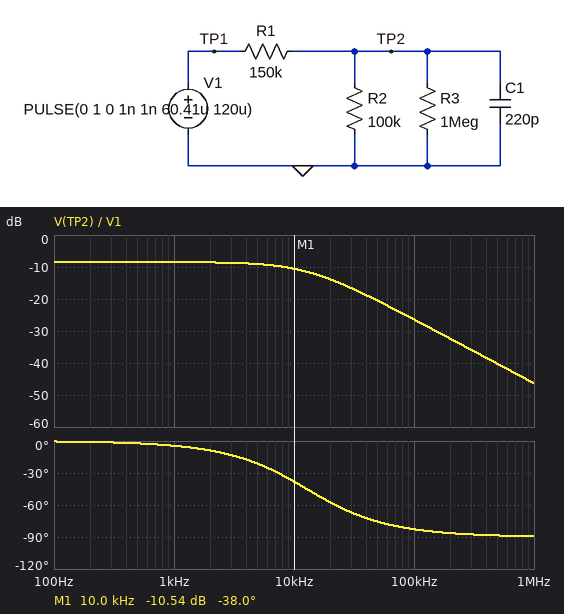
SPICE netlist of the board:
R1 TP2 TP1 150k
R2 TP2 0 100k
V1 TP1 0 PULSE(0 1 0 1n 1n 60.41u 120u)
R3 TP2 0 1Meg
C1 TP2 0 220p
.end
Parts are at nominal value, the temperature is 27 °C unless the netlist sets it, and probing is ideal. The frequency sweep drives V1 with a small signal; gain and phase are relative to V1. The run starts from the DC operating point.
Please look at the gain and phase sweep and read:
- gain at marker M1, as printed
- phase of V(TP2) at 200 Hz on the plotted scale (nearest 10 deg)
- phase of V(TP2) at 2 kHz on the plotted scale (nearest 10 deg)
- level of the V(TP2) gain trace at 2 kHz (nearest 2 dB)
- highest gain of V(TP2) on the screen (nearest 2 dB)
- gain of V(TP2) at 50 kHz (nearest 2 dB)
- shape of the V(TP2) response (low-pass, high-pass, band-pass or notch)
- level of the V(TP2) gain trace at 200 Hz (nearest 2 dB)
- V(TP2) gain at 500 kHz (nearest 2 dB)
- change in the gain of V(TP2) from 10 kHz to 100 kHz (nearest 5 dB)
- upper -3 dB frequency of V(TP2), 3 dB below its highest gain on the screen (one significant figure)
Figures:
-10.54 dB
0 deg
-10 deg
-8 dB
-8 dB
-20 dB
low-pass
-8 dB
-40 dB
-15 dB
10 kHz
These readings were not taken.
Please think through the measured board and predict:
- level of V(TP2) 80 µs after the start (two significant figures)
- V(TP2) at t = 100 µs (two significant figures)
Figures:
78 mV
16 mV
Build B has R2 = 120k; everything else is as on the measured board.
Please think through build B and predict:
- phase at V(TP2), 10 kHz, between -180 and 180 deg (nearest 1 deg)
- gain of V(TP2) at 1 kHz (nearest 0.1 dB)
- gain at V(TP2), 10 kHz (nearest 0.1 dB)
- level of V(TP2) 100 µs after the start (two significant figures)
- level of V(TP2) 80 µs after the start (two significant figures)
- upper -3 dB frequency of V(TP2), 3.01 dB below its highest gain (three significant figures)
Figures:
-41 deg
-7.6 dB
-10.0 dB
23 mV
99 mV
11.6 kHz
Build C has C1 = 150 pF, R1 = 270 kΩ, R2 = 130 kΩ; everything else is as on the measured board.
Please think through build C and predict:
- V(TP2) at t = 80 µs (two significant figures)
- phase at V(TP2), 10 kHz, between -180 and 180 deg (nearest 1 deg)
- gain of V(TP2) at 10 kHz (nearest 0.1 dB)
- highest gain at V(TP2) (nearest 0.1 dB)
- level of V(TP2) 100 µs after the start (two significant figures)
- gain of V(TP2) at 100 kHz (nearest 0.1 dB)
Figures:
59 mV
-37 deg
-12.5 dB
-10.5 dB
11 mV
-28.2 dB
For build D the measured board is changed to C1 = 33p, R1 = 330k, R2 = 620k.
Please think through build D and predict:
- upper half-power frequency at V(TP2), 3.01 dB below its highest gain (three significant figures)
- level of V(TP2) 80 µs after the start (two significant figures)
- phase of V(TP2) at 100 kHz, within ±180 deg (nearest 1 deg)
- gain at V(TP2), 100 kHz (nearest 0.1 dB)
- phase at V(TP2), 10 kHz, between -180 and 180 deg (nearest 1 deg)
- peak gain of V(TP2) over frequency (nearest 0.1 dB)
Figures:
27.2 kHz
19 mV
-75 deg
-17.0 dB
-20 deg
-5.4 dB
